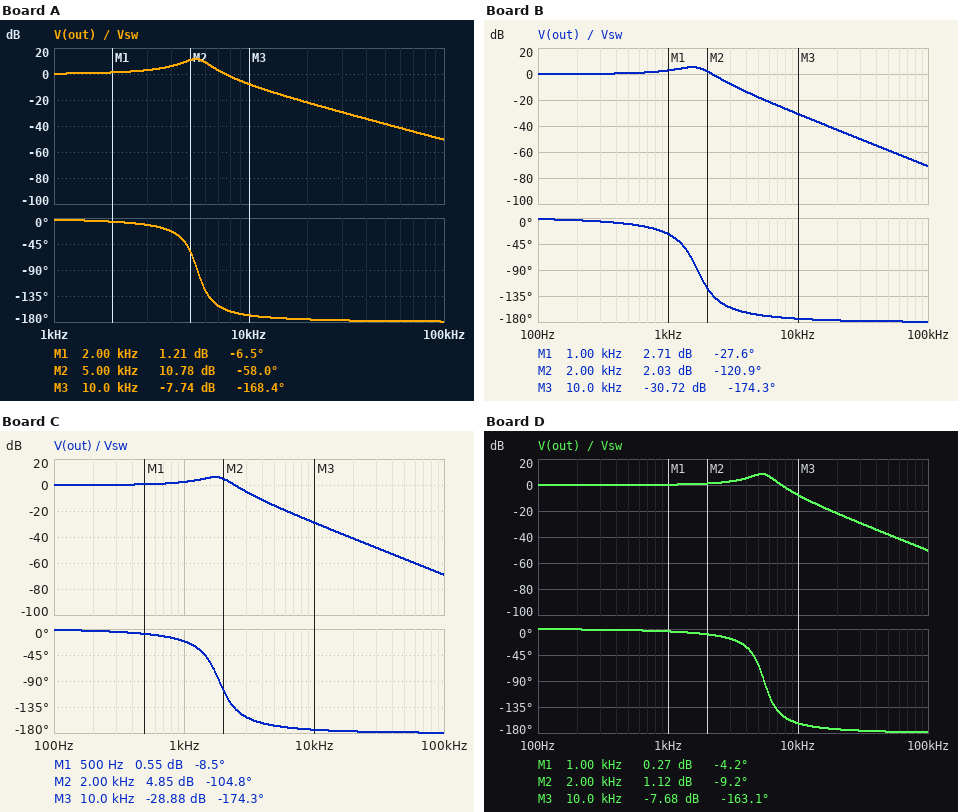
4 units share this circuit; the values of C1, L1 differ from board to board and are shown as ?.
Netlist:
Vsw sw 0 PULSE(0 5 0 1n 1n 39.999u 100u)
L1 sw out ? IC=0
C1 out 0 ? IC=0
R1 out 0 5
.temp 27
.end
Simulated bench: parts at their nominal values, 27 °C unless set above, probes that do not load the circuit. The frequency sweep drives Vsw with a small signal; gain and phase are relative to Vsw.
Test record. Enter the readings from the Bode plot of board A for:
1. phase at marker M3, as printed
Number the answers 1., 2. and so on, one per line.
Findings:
1. -168.4 deg
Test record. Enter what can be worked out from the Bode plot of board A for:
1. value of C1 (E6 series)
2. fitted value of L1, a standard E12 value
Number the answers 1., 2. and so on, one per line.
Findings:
1. 22 µF
2. 39 µH
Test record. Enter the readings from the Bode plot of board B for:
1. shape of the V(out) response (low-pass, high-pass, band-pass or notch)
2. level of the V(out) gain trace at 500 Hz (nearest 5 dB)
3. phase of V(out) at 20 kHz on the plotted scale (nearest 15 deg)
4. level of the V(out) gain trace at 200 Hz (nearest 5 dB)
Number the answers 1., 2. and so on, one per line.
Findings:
1. low-pass
2. 0 dB
3. -180 deg
4. 0 dB
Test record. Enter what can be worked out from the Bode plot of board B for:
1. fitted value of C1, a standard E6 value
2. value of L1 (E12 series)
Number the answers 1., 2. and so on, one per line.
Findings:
1. 33 µF
2. 270 µH
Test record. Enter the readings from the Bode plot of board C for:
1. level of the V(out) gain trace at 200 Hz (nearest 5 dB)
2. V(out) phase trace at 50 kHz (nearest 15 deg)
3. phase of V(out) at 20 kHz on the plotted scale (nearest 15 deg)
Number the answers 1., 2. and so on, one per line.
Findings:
1. 0 dB
2. -180 deg
3. -180 deg
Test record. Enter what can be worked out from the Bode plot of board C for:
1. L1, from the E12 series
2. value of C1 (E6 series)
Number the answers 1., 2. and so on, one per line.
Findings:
1. 220 µH
2. 33 µF
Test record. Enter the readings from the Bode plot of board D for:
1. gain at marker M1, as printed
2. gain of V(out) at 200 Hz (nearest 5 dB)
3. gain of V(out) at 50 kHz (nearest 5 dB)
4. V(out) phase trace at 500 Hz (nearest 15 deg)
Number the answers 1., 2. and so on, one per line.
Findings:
1. 0.27 dB
2. 0 dB
3. -40 dB
4. 0 deg
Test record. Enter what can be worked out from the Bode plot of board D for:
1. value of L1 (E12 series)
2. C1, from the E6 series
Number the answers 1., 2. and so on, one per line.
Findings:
1. 56 µH
2. 15 µF
